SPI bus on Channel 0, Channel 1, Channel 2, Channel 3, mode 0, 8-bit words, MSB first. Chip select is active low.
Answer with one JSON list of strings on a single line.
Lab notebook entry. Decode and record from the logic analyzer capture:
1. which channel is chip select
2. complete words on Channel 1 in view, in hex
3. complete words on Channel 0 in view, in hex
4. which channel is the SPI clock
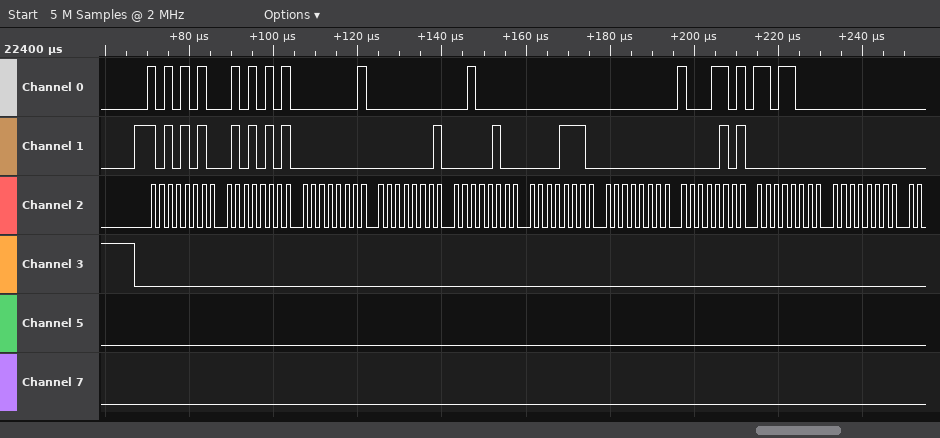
["Channel 3", "AA, 55, 00, 01, 04, 0E, 00, 05, 00, 00", "AA, 55, 01, 00, 20, 00, 00, 8D, D8, 00", "Channel 2"]
